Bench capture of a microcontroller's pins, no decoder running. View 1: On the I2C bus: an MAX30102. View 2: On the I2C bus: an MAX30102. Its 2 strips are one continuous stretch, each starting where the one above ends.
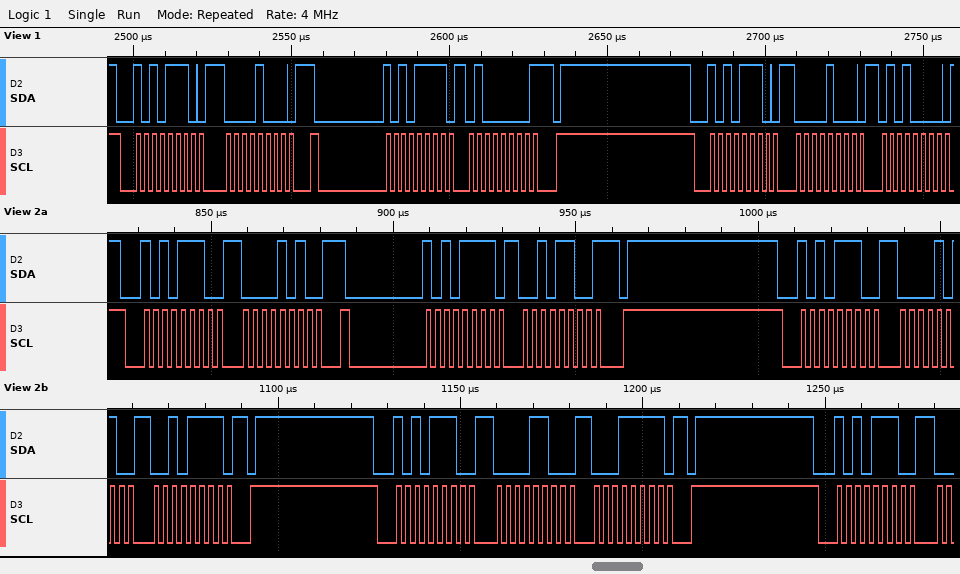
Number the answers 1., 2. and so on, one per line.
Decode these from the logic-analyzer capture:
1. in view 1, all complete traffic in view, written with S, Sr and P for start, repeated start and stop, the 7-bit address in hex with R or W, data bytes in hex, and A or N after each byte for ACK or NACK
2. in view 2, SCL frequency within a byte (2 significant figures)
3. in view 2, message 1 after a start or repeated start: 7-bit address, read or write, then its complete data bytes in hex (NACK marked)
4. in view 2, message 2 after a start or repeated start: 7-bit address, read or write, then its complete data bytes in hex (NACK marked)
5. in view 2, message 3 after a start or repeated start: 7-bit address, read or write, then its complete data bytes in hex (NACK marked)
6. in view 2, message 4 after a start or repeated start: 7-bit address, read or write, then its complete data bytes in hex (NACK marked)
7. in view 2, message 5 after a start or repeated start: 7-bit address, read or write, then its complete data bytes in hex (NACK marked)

1. S 57W A 08 A Sr 57R A 40 N P S 57W A 08 A 50 A
2. 400 kHz
3. 0x57 write: 0A
4. 0x57 read: 2C NACK
5. 0x57 write: 0A 2F
6. 0x57 write: 0C 1F
7. 0x57 write
